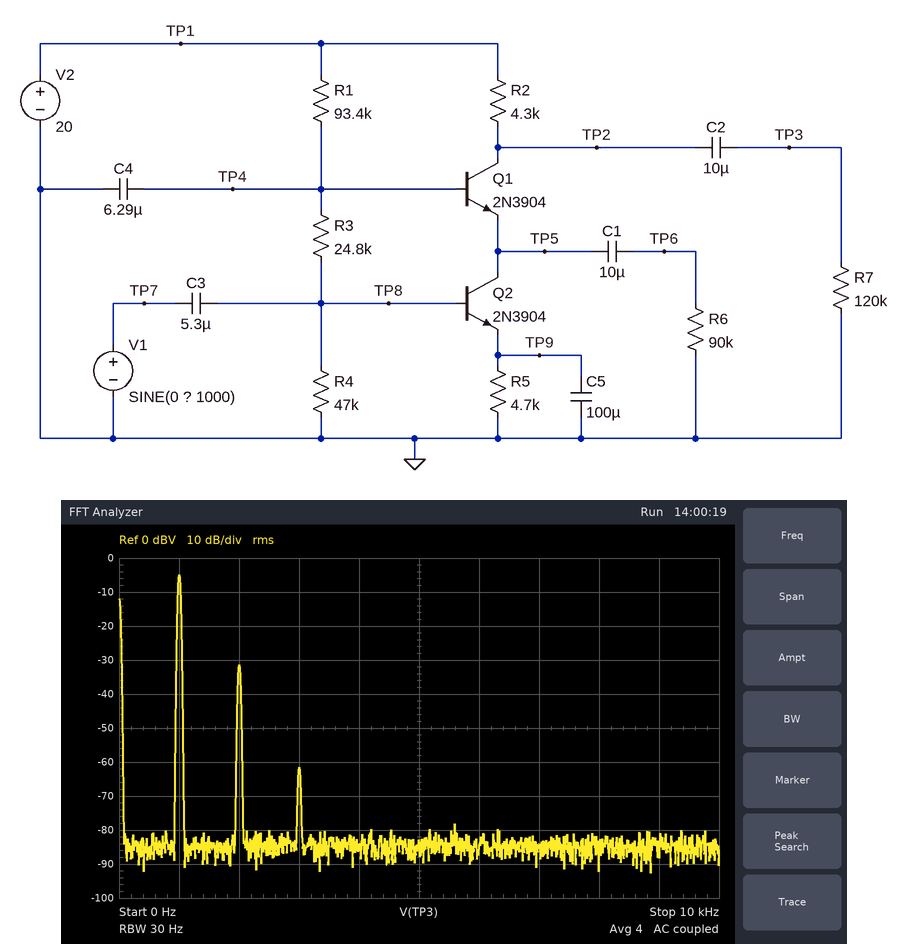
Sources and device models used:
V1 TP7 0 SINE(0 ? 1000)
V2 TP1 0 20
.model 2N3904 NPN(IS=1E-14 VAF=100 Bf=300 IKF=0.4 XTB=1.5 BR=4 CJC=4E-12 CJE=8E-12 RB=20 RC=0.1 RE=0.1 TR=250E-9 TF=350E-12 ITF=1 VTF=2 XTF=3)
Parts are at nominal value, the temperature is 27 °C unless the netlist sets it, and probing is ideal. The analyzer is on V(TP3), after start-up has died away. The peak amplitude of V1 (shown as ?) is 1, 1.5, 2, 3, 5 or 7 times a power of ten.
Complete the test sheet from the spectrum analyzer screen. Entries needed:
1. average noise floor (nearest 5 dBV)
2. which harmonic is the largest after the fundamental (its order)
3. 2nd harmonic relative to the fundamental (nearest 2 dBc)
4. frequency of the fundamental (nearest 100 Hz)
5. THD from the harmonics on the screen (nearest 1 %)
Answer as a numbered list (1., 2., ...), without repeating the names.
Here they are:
1. -85 dBV
2. 2
3. -26 dBc
4. 1.0 kHz
5. 5 %
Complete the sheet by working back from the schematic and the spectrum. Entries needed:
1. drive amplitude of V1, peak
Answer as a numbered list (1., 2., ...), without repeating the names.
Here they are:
1. 5 mV
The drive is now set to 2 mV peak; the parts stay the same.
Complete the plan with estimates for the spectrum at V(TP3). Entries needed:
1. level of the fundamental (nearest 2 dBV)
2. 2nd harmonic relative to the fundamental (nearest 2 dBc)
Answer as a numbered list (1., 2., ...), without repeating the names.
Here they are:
1. -12 dBV
2. -34 dBc
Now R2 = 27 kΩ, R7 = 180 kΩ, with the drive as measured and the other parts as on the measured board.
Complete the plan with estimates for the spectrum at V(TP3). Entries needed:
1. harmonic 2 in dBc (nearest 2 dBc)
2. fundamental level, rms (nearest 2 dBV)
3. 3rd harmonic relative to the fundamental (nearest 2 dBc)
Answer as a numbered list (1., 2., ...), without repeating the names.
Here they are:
1. -4 dBc
2. -10 dBV
3. -10 dBc
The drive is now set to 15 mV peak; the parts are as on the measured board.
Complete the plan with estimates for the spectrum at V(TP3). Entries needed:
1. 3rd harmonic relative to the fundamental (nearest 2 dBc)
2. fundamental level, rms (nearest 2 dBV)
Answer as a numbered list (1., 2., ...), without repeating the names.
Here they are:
1. -38 dBc
2. 4 dBV
